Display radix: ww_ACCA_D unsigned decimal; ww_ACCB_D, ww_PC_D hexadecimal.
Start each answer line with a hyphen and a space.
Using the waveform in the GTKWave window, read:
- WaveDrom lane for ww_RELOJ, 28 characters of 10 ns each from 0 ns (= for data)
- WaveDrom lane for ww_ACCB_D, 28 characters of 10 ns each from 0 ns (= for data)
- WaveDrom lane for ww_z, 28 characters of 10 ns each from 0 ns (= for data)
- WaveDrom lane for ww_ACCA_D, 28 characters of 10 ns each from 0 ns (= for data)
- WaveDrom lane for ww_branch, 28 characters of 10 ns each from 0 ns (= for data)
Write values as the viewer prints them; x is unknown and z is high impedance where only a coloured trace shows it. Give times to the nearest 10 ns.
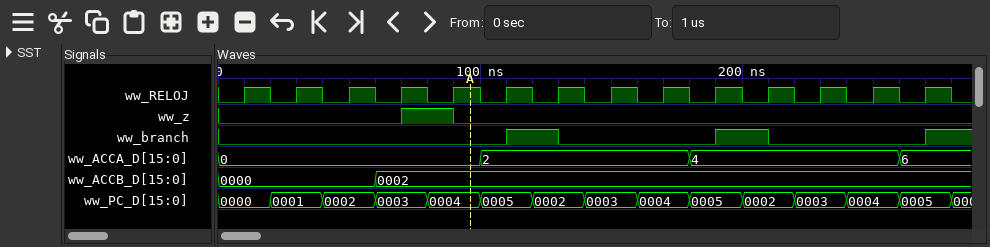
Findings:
- {name: 'ww_RELOJ', wave: '0101010101010101010101010101'}
- {name: 'ww_ACCB_D', wave: '=.....=.....................', data: '0000 0002'}
- {name: 'ww_z', wave: '0......1.0..................'}
- {name: 'ww_ACCA_D', wave: '=.........=.......=.......=.', data: '0 2 4 6'}
- {name: 'ww_branch', wave: '0..........1.0.....1.0.....1'}
